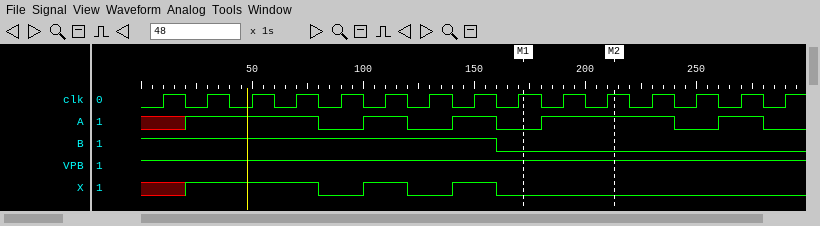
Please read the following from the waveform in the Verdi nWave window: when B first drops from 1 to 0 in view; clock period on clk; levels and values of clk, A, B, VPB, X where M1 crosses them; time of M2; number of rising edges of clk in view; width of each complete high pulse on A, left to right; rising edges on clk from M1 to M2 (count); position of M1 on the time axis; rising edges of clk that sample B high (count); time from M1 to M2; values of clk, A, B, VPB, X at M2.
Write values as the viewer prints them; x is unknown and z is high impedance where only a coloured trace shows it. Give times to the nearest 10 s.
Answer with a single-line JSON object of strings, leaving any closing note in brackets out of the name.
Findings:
{"when B first drops from 1 to 0 in view": "160 s", "clock period on clk": "20 s", "levels and values of clk, A, B, VPB, X where M1 crosses them": "clk=1, A=0, B=0, VPB=1, X=0", "time of M2": "210 s", "number of rising edges of clk in view": "15", "width of each complete high pulse on A, left to right": "20 s, 20 s, 60 s, 20 s", "rising edges on clk from M1 to M2": "2", "position of M1 on the time axis": "170 s", "rising edges of clk that sample B high": "8", "time from M1 to M2": "40 s", "values of clk, A, B, VPB, X at M2": "clk=1, A=1, B=0, VPB=1, X=0"}
